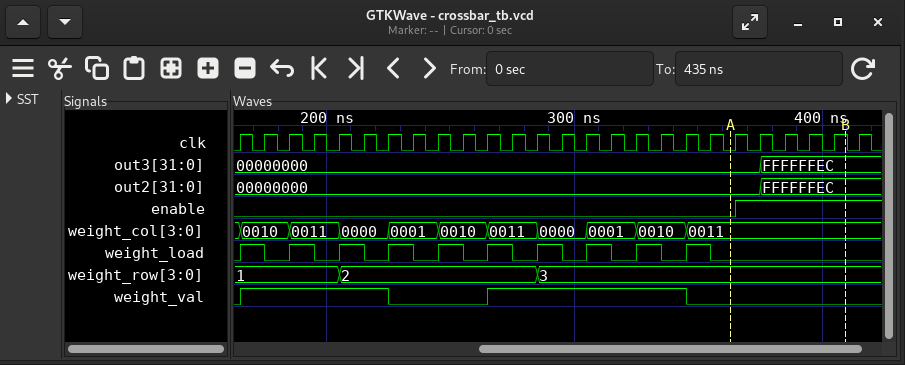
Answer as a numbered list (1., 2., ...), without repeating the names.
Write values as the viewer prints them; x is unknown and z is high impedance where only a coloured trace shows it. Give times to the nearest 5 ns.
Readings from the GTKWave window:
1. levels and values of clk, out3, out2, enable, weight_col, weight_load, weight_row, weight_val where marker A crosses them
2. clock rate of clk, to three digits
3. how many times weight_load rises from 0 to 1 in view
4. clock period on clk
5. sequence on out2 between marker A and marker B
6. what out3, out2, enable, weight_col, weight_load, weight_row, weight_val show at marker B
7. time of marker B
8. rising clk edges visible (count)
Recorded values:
1. clk=0, out3=00000000, out2=00000000, enable=0, weight_col=0011, weight_load=0, weight_row=3, weight_val=0
2. 100 MHz
3. 10
4. 10 ns
5. 00000000, FFFFFFEC
6. out3=FFFFFFEC, out2=FFFFFFEC, enable=1, weight_col=0011, weight_load=0, weight_row=3, weight_val=0
7. 410 ns
8. 26
